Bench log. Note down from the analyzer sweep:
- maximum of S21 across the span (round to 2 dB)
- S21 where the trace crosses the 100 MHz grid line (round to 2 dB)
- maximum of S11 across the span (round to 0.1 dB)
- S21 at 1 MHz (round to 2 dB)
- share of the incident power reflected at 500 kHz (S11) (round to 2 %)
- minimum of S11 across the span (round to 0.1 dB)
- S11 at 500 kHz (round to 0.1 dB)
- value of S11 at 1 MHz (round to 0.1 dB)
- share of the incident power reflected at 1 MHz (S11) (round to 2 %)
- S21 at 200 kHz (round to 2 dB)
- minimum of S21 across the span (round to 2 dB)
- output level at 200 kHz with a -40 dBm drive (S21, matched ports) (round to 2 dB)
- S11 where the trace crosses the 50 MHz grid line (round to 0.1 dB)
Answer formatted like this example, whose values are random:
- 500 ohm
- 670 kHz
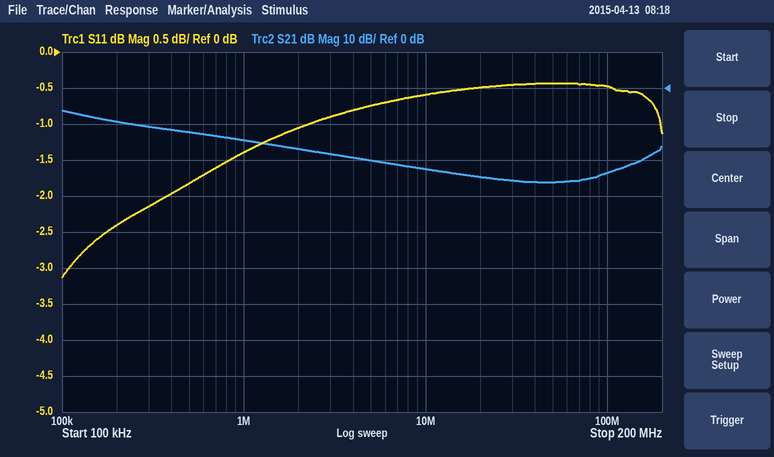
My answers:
- -6 dB
- -24 dB
- -0.4 dB
- -14 dB
- 66 %
- -3.1 dB
- -1.8 dB
- -1.4 dB
- 72 %
- -10 dB
- -26 dB
- -50 dBm
- -0.4 dB
